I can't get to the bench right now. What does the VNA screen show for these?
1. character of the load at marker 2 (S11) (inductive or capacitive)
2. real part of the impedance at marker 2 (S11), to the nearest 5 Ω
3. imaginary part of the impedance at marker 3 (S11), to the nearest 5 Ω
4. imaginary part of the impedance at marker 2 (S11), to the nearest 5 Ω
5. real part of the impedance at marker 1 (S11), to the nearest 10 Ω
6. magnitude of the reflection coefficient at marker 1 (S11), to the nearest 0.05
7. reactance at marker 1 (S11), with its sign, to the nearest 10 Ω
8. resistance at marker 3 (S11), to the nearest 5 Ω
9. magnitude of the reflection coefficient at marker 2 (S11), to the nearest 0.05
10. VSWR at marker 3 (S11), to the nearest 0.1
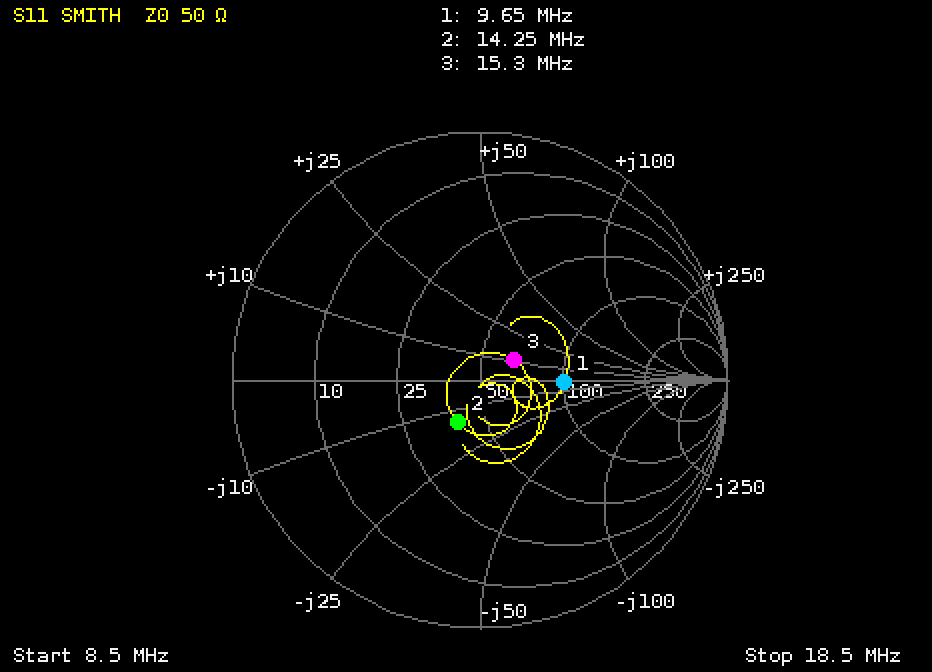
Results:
capacitive
40 Ω
+10 Ω
-15 Ω
100 Ω
0.35
0 Ω
65 Ω
0.20
1.4
